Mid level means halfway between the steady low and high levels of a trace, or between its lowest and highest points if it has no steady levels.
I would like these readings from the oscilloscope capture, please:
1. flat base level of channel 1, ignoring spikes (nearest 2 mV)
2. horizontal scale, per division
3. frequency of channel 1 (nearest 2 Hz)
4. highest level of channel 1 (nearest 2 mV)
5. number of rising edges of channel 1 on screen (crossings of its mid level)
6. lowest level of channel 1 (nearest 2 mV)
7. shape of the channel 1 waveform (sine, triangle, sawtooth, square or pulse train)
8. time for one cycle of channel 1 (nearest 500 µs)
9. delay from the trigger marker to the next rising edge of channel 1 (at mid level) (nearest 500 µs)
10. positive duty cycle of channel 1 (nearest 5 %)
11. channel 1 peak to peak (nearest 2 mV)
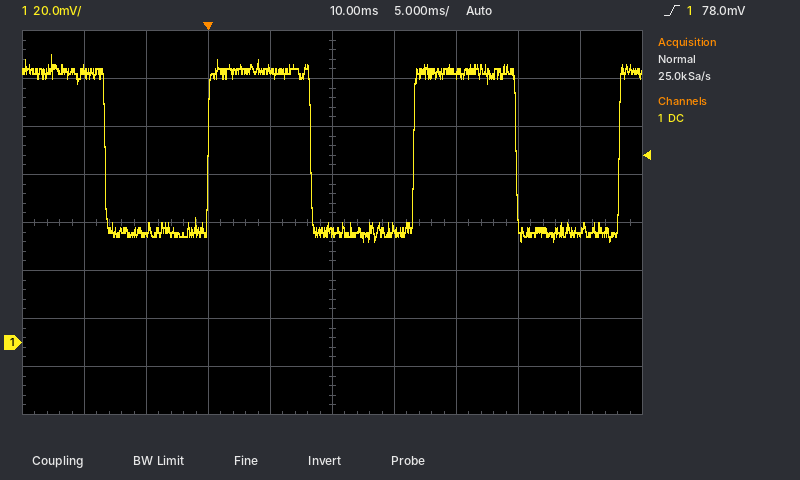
46 mV
5 ms
60 Hz
120 mV
3
42 mV
square
16.5 ms
16.5 ms
50 %
78 mV
